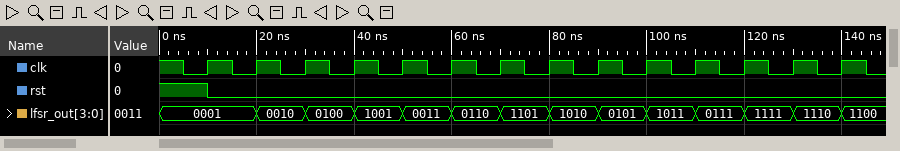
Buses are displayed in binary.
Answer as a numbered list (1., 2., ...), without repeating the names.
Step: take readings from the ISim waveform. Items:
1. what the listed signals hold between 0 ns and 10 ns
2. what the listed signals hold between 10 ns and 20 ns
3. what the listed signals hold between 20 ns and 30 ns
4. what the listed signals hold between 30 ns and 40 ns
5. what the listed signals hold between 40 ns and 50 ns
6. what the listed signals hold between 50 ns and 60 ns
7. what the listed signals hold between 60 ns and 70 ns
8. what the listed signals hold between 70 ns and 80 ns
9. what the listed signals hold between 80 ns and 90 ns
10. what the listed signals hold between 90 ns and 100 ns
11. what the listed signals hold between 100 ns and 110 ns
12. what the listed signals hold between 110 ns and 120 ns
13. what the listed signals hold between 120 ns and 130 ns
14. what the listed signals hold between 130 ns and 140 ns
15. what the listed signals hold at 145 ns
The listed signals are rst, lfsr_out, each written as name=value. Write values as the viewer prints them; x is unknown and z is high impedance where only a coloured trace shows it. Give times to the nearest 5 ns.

1. rst=1, lfsr_out=0001
2. rst=0, lfsr_out=0001
3. rst=0, lfsr_out=0010
4. rst=0, lfsr_out=0100
5. rst=0, lfsr_out=1001
6. rst=0, lfsr_out=0011
7. rst=0, lfsr_out=0110
8. rst=0, lfsr_out=1101
9. rst=0, lfsr_out=1010
10. rst=0, lfsr_out=0101
11. rst=0, lfsr_out=1011
12. rst=0, lfsr_out=0111
13. rst=0, lfsr_out=1111
14. rst=0, lfsr_out=1110
15. rst=0, lfsr_out=1100
